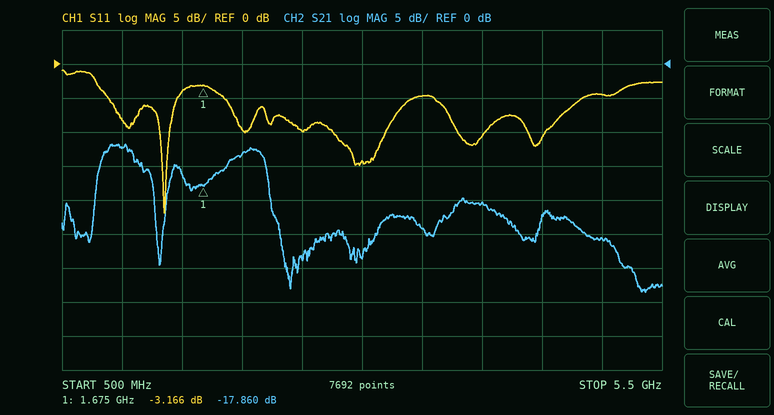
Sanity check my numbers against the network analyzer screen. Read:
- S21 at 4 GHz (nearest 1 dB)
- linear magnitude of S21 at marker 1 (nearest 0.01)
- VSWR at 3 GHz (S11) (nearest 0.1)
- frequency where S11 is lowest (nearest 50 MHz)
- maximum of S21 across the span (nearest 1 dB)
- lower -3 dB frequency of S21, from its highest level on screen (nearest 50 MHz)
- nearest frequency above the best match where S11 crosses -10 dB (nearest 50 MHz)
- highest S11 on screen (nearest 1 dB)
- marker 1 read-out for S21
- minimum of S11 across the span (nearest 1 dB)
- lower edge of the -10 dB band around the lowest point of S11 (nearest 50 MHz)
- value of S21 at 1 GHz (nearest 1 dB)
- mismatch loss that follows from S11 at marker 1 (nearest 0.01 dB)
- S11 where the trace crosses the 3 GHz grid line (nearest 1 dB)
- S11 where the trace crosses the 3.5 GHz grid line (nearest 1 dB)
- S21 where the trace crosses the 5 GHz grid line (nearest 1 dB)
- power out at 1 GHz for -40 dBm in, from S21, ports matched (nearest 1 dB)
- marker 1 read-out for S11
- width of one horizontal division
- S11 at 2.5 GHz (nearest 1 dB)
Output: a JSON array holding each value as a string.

["-20 dB", "0.13", "1.5", "1.35 GHz", "-12 dB", "800 MHz", "1.40 GHz", "-1 dB", "-17.860 dB", "-22 dB", "1.30 GHz", "-12 dB", "2.86 dB", "-14 dB", "-5 dB", "-26 dB", "-52 dBm", "-3.166 dB", "500 MHz", "-10 dB"]
